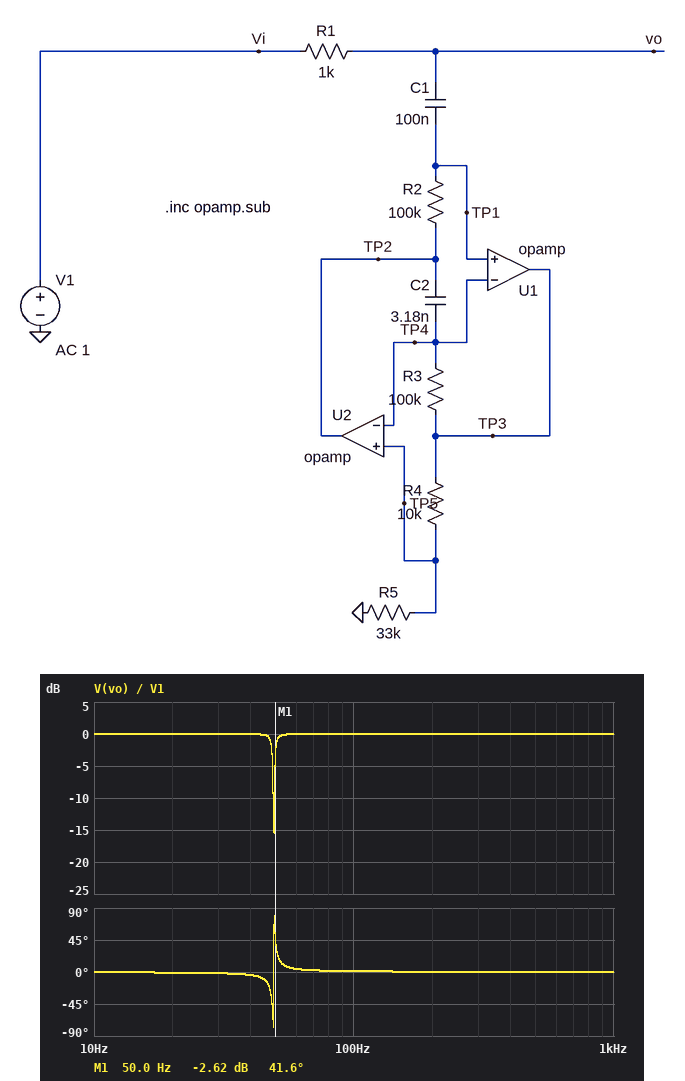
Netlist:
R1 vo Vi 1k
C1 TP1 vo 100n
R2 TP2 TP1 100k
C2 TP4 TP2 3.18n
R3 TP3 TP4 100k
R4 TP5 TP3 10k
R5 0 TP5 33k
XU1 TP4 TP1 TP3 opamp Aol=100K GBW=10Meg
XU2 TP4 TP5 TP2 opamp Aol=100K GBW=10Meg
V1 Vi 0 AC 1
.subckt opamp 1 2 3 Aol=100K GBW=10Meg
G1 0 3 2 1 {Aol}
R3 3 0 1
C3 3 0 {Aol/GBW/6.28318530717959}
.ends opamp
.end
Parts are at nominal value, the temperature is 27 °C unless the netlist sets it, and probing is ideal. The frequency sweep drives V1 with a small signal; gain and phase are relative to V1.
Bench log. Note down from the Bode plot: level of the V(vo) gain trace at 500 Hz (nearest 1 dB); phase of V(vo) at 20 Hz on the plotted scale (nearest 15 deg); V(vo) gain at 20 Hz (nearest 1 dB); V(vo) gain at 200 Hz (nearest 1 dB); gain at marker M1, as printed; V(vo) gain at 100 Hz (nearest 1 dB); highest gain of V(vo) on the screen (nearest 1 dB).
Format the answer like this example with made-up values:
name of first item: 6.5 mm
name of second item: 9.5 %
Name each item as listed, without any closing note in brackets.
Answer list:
level of the V(vo) gain trace at 500 Hz: 0 dB
phase of V(vo) at 20 Hz on the plotted scale: 0 deg
V(vo) gain at 20 Hz: 0 dB
V(vo) gain at 200 Hz: 0 dB
gain at marker M1, as printed: -2.62 dB
V(vo) gain at 100 Hz: 0 dB
highest gain of V(vo) on the screen: 0 dB
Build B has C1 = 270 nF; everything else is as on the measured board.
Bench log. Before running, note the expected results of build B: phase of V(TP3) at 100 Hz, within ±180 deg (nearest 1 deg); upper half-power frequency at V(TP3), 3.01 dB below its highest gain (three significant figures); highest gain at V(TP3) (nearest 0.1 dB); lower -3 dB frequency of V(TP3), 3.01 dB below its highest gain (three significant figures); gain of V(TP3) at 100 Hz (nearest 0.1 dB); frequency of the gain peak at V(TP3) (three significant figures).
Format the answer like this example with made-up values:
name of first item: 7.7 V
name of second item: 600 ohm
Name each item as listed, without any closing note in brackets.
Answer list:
phase of V(TP3) at 100 Hz, within ±180 deg: 1 deg
upper half-power frequency at V(TP3), 3.01 dB below its highest gain: 30.7 Hz
highest gain at V(TP3): 28.2 dB
lower -3 dB frequency of V(TP3), 3.01 dB below its highest gain: 29.2 Hz
gain of V(TP3) at 100 Hz: 3.1 dB
frequency of the gain peak at V(TP3): 29.9 Hz
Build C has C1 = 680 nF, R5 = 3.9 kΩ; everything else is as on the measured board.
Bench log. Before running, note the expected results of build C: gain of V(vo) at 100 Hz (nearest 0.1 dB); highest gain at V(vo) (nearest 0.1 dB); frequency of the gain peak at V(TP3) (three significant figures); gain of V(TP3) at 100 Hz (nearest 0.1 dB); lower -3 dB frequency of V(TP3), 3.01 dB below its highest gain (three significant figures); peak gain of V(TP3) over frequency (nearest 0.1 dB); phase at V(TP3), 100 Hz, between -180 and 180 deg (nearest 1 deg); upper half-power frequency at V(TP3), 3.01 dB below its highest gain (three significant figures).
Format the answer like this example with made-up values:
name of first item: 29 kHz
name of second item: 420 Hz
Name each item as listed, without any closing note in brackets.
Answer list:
gain of V(vo) at 100 Hz: -0.1 dB
highest gain at V(vo): 0 dB
frequency of the gain peak at V(TP3): 55.6 Hz
gain of V(TP3) at 100 Hz: 14.0 dB
lower -3 dB frequency of V(TP3), 3.01 dB below its highest gain: 49.9 Hz
peak gain of V(TP3) over frequency: 23.7 dB
phase at V(TP3), 100 Hz, between -180 and 180 deg: 10 deg
upper half-power frequency at V(TP3), 3.01 dB below its highest gain: 63.7 Hz
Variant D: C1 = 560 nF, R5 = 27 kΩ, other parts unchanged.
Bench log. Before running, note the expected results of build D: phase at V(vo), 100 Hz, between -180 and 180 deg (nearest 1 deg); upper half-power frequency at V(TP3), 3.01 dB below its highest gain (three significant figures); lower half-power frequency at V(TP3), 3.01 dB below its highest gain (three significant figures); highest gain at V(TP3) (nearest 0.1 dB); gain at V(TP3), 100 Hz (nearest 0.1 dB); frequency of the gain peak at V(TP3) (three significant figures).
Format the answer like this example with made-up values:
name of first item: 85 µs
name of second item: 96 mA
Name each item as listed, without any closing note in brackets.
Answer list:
phase at V(vo), 100 Hz, between -180 and 180 deg: 1 deg
upper half-power frequency at V(TP3), 3.01 dB below its highest gain: 24.0 Hz
lower half-power frequency at V(TP3), 3.01 dB below its highest gain: 22.1 Hz
highest gain at V(TP3): 24.6 dB
gain at V(TP3), 100 Hz: 3.2 dB
frequency of the gain peak at V(TP3): 23.0 Hz
